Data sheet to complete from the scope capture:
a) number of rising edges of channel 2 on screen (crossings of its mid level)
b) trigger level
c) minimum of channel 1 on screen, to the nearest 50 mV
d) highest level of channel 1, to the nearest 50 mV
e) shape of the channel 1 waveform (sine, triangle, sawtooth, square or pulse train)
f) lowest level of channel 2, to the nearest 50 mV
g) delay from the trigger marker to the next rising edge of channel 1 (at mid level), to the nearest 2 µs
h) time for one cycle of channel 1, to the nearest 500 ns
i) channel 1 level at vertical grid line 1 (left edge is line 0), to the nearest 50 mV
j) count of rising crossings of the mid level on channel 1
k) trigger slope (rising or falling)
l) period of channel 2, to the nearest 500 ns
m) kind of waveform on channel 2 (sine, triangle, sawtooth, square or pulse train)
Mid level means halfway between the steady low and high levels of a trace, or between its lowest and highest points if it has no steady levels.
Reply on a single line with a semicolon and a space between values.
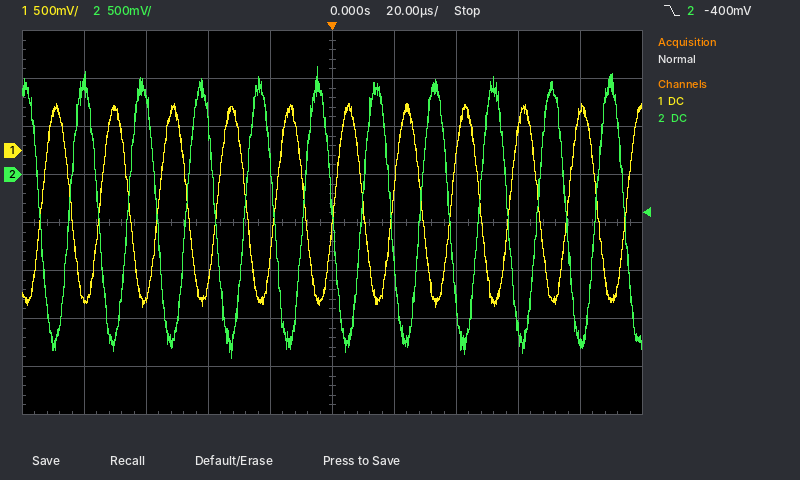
10; -400 mV; -1.65 V; 500 mV; sine; -1.90 V; 20 µs; 19.0 µs; -1.55 V; 11; falling; 19.0 µs; sine
